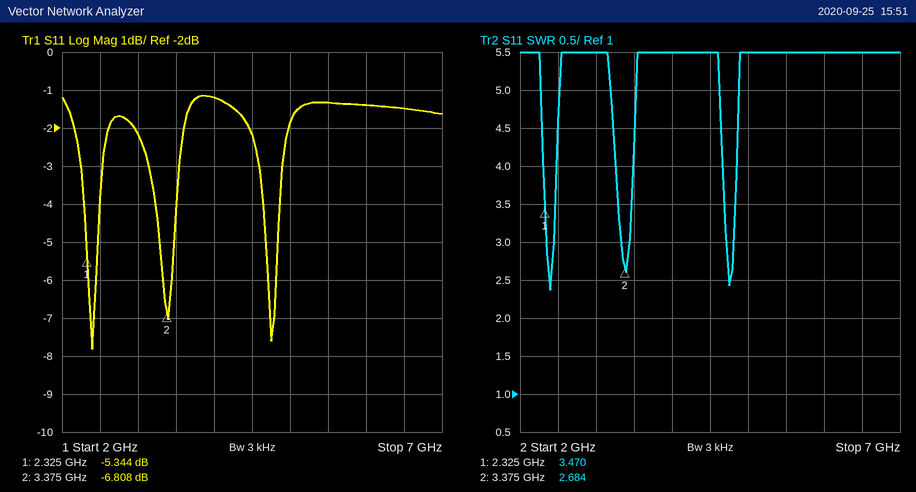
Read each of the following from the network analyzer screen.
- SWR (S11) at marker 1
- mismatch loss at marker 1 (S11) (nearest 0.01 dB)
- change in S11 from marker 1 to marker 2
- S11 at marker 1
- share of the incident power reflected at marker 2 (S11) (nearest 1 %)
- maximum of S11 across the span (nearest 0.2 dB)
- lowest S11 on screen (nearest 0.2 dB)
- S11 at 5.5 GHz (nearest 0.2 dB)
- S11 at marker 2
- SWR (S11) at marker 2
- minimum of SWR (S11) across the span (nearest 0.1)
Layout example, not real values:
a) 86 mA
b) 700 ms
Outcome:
a) 3.470
b) 1.50 dB
c) -1.464 dB
d) -5.344 dB
e) 21 %
f) -1.2 dB
g) -7.8 dB
h) -1.4 dB
i) -6.808 dB
j) 2.684
k) 2.4
